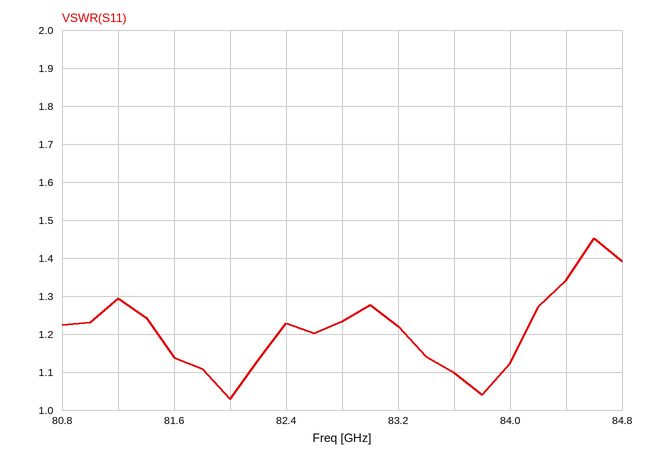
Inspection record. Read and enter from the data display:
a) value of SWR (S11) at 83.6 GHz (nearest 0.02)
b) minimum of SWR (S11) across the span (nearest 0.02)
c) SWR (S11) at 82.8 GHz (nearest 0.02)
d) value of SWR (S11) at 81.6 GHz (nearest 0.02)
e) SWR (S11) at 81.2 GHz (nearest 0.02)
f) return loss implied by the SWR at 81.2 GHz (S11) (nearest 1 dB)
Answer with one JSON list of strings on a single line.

["1.10", "1.02", "1.24", "1.14", "1.30", "18 dB"]
